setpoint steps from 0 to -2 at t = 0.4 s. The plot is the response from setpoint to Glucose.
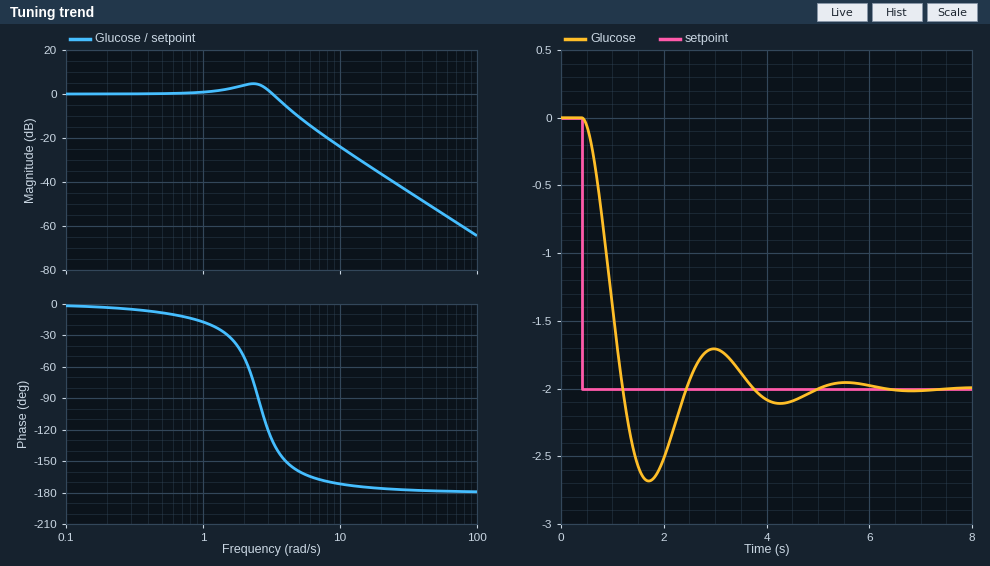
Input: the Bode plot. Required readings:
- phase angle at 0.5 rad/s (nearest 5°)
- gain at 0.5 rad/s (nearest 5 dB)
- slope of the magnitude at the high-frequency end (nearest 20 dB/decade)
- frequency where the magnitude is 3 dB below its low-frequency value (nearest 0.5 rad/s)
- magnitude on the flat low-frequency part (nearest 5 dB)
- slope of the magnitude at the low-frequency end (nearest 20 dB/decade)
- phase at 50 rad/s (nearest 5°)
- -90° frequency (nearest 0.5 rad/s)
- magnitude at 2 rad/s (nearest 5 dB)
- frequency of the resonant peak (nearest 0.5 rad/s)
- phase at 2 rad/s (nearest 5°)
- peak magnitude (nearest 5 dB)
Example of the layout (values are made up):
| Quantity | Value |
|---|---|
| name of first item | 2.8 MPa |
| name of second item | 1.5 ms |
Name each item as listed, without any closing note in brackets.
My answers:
| Quantity | Value |
|---|---|
| phase angle at 0.5 rad/s | -10° |
| gain at 0.5 rad/s | 0 dB |
| slope of the magnitude at the high-frequency end | -40 dB/decade |
| frequency where the magnitude is 3 dB below its low-frequency value | 3.5 rad/s |
| magnitude on the flat low-frequency part | 0 dB |
| slope of the magnitude at the low-frequency end | 0 dB/decade |
| phase at 50 rad/s | -180° |
| -90° frequency | 2.5 rad/s |
| magnitude at 2 rad/s | 5 dB |
| frequency of the resonant peak | 2.5 rad/s |
| phase at 2 rad/s | -50° |
| peak magnitude | 5 dB |
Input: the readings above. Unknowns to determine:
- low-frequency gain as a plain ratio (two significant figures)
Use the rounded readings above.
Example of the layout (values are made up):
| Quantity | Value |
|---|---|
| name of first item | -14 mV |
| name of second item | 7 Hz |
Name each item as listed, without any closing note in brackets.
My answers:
| Quantity | Value |
|---|---|
| low-frequency gain as a plain ratio | 1.0 |
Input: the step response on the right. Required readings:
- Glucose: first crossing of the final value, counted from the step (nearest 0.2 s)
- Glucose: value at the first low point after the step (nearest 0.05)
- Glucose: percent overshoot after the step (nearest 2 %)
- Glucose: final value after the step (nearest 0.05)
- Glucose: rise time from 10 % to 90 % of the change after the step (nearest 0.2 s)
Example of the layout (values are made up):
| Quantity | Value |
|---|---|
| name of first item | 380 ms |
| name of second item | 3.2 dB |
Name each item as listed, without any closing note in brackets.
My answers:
| Quantity | Value |
|---|---|
| Glucose: first crossing of the final value, counted from the step | 0.8 s |
| Glucose: value at the first low point after the step | -2.70 |
| Glucose: percent overshoot after the step | 34 % |
| Glucose: final value after the step | -2.00 |
| Glucose: rise time from 10 % to 90 % of the change after the step | 0.6 s |
